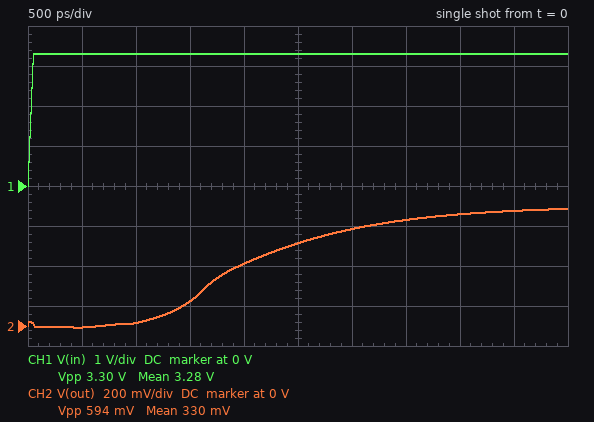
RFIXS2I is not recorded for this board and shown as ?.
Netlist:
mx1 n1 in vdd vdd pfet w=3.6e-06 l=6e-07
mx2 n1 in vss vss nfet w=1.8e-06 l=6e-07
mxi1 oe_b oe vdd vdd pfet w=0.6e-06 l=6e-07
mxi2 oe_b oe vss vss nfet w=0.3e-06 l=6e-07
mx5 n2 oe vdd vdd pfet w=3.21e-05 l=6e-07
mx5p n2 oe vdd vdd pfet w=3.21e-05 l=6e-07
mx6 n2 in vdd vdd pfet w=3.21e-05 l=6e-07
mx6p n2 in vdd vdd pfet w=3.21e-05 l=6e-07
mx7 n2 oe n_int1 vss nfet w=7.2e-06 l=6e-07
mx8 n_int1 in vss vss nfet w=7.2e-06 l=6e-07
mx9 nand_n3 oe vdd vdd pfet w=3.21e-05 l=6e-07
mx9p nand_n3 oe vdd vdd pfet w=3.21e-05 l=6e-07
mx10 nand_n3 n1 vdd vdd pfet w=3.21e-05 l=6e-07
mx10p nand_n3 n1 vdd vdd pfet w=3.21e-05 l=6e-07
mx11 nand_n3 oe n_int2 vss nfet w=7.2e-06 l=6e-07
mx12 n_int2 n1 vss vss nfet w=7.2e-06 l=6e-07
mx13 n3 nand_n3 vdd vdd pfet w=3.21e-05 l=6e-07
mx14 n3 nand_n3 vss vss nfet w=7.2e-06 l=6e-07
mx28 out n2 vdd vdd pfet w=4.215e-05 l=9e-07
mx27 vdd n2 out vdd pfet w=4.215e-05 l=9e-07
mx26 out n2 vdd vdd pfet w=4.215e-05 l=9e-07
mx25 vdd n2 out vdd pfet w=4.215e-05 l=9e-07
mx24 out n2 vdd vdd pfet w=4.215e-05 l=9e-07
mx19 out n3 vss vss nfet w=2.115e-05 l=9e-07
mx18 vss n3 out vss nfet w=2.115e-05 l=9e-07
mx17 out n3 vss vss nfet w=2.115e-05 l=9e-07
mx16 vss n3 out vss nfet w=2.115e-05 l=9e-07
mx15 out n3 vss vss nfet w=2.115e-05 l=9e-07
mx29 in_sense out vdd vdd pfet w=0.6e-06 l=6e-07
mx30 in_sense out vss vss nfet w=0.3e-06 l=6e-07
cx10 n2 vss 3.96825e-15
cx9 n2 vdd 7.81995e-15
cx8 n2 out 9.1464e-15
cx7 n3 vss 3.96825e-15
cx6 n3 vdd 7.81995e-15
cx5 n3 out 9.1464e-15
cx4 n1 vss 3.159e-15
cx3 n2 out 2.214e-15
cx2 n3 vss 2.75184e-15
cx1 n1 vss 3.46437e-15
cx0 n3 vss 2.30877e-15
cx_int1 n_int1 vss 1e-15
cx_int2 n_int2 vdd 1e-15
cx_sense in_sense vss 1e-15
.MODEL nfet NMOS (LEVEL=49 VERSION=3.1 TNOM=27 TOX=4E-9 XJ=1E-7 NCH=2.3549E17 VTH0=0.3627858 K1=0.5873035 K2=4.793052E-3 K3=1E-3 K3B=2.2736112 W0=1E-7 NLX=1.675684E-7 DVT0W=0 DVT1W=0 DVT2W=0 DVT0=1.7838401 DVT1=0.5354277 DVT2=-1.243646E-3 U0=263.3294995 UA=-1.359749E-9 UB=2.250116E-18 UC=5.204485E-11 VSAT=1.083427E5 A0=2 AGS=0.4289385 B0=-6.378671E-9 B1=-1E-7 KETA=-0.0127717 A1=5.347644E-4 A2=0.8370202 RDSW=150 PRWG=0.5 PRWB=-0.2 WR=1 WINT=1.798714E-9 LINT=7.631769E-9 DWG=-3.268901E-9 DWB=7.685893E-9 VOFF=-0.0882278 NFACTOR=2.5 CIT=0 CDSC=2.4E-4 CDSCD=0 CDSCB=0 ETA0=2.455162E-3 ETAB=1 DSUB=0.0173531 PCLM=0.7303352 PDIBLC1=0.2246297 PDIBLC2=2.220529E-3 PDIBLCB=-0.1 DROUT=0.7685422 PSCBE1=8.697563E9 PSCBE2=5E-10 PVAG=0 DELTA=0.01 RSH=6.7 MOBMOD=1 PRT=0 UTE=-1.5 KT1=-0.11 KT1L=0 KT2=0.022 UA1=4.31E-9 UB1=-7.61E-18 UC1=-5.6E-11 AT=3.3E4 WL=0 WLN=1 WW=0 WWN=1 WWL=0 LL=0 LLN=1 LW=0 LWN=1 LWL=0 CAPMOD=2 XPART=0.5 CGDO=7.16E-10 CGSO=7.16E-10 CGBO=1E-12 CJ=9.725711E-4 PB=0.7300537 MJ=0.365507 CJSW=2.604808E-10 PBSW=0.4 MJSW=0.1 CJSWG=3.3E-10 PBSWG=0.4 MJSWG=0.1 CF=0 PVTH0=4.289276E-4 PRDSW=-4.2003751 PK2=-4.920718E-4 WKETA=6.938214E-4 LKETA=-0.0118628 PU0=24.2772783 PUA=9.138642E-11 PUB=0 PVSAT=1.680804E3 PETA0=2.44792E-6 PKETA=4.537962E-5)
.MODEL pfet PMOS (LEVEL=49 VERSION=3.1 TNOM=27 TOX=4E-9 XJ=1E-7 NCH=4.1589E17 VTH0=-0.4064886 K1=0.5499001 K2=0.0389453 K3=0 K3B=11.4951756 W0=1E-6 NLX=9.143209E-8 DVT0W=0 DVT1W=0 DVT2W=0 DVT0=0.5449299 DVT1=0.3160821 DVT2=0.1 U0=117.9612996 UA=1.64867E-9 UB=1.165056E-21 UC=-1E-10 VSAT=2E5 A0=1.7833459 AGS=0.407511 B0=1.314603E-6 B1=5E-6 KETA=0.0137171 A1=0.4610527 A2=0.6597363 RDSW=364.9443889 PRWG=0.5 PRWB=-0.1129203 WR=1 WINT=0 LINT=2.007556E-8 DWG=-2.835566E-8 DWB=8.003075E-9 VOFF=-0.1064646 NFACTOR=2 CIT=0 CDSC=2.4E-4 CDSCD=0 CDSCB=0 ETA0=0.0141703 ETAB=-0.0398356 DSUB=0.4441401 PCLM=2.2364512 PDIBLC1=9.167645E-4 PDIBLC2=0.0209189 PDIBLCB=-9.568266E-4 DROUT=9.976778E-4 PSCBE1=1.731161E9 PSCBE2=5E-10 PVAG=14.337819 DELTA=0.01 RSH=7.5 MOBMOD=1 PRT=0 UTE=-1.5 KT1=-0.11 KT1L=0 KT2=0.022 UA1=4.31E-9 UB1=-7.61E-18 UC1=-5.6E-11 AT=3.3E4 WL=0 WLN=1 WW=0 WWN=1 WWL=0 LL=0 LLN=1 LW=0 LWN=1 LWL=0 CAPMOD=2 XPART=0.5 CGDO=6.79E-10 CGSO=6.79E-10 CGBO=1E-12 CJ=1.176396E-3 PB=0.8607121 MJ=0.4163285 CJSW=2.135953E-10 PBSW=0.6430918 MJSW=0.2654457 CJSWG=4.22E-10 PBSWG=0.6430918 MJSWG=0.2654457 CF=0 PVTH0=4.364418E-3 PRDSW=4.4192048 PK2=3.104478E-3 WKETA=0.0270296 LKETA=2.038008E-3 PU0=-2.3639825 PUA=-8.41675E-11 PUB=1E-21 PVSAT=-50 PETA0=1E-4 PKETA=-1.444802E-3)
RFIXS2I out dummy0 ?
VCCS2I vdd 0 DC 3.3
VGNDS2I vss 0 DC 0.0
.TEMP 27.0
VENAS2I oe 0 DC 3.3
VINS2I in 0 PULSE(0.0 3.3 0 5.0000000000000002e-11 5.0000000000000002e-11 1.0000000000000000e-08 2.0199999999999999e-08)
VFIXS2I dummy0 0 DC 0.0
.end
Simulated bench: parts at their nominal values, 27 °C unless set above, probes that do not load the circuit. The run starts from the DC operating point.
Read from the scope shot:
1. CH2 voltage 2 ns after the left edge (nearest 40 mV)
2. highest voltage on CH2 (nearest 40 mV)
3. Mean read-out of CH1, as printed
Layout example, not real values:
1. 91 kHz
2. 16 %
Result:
1. 320 mV
2. 600 mV
3. 3.28 V
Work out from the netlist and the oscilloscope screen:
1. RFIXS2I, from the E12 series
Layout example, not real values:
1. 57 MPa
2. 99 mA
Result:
1. 18 Ω
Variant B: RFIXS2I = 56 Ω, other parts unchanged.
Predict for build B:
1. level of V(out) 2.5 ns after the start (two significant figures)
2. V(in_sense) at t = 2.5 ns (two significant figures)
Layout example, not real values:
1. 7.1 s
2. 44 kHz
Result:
1. 1.2 V
2. 2.9 V
